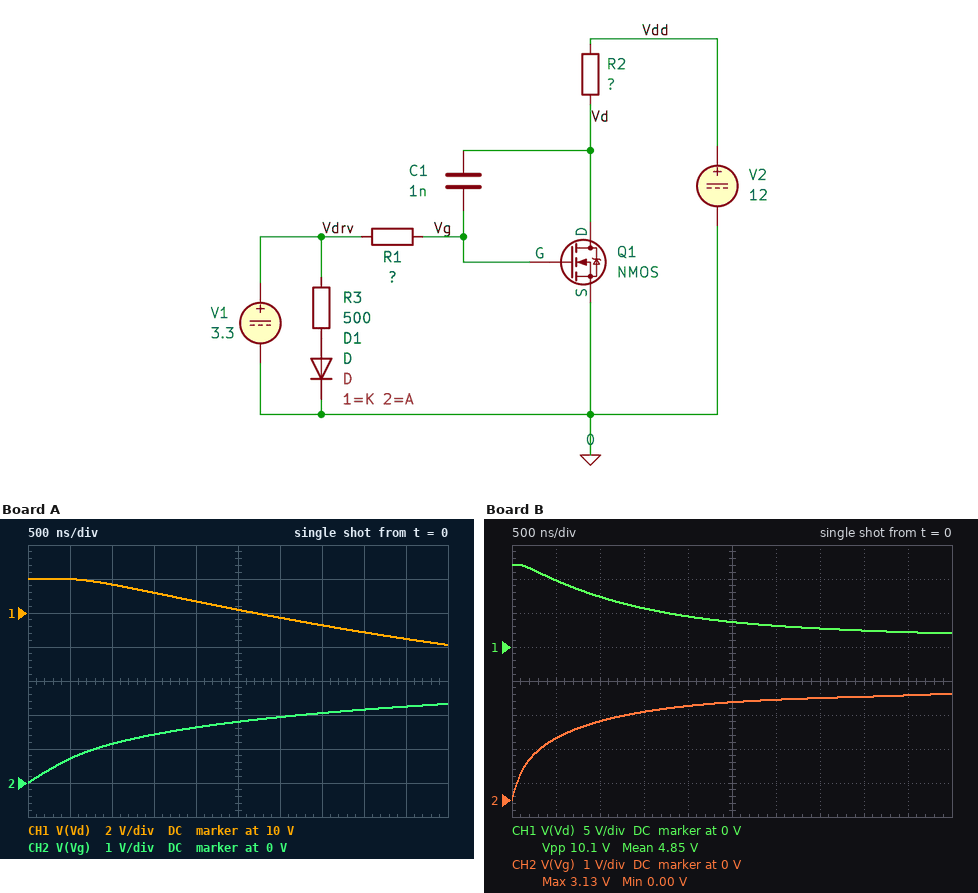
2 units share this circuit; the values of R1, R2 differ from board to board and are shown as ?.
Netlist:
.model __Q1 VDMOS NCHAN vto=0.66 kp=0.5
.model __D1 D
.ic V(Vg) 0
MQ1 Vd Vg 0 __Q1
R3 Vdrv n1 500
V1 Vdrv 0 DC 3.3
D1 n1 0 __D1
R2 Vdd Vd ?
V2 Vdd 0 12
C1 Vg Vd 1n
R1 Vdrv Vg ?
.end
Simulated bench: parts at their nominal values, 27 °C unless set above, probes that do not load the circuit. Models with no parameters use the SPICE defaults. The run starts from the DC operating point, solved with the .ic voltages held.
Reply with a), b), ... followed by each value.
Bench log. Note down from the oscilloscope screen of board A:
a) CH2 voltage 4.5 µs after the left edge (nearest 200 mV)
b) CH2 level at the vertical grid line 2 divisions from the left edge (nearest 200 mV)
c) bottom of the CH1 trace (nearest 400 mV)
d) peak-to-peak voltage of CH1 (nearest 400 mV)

a) 2.2 V
b) 1.2 V
c) 8.0 V
d) 4.0 V
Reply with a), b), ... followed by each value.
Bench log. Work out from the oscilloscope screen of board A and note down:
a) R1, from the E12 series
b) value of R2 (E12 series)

a) 820 Ω
b) 5.6 Ω
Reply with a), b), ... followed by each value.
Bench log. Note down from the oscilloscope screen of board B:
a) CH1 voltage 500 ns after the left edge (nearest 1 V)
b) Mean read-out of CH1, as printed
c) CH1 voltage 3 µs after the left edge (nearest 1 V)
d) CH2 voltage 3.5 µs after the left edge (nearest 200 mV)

a) 10 V
b) 4.85 V
c) 3 V
d) 3.0 V
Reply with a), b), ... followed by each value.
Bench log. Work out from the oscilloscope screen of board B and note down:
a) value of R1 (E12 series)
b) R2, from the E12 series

a) 150 Ω
b) 6.8 Ω
